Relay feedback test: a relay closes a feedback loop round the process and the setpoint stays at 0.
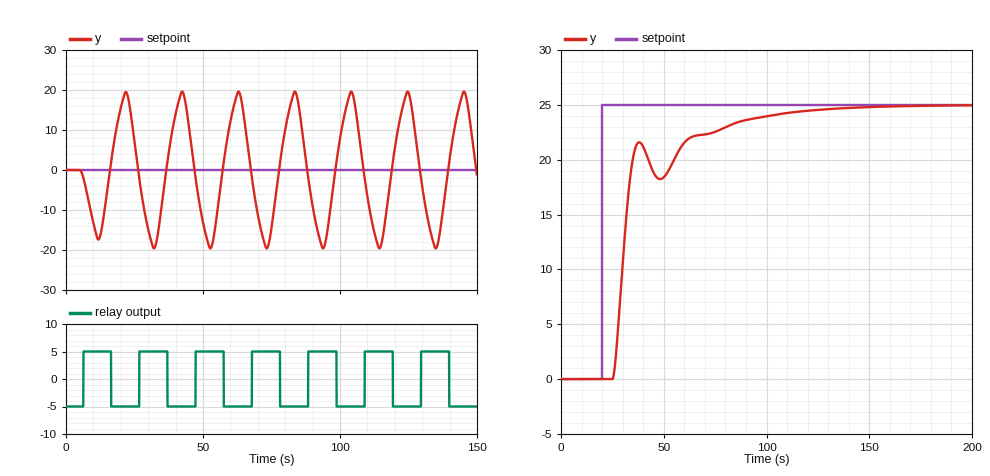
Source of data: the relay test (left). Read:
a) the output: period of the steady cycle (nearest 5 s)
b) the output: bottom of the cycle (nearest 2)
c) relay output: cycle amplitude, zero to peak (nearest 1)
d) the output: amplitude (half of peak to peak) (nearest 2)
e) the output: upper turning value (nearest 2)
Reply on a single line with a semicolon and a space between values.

20 s; -20; 5; 20; 20
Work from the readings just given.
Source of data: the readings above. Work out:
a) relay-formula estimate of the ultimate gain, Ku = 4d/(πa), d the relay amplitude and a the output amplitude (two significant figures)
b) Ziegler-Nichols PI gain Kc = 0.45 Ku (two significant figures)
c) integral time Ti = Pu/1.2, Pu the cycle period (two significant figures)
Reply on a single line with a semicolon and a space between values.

0.32; 0.14; 17 s
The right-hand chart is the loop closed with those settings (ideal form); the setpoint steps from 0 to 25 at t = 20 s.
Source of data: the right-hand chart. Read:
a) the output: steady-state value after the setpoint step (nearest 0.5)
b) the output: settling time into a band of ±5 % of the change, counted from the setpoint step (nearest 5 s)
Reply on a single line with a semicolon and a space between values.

25.0; 75 s
